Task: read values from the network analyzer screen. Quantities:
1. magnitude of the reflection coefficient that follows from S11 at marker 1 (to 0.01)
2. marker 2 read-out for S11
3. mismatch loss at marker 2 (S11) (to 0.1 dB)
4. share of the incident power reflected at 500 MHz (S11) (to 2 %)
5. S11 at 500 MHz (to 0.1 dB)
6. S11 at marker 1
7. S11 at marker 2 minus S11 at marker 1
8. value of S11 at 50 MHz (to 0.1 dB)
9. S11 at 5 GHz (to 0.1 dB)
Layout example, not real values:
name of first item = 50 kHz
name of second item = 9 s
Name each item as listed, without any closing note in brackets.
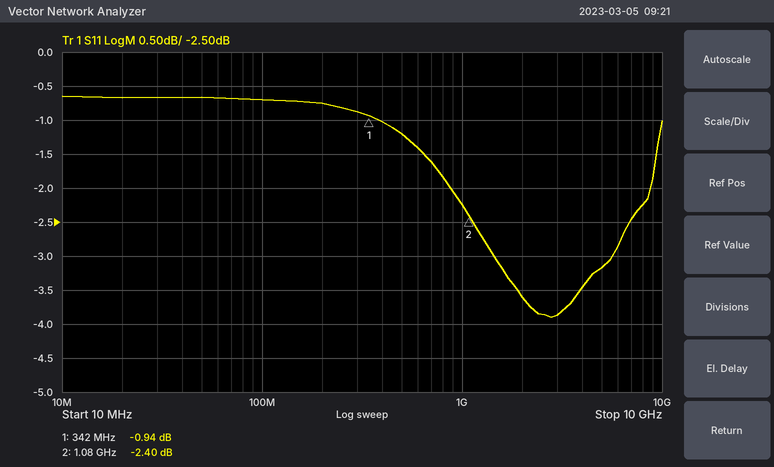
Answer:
magnitude of the reflection coefficient that follows from S11 at marker 1 = 0.90
marker 2 read-out for S11 = -2.40 dB
mismatch loss at marker 2 (S11) = 3.7 dB
share of the incident power reflected at 500 MHz (S11) = 76 %
S11 at 500 MHz = -1.2 dB
S11 at marker 1 = -0.94 dB
S11 at marker 2 minus S11 at marker 1 = -1.46 dB
value of S11 at 50 MHz = -0.7 dB
S11 at 5 GHz = -3.2 dB
